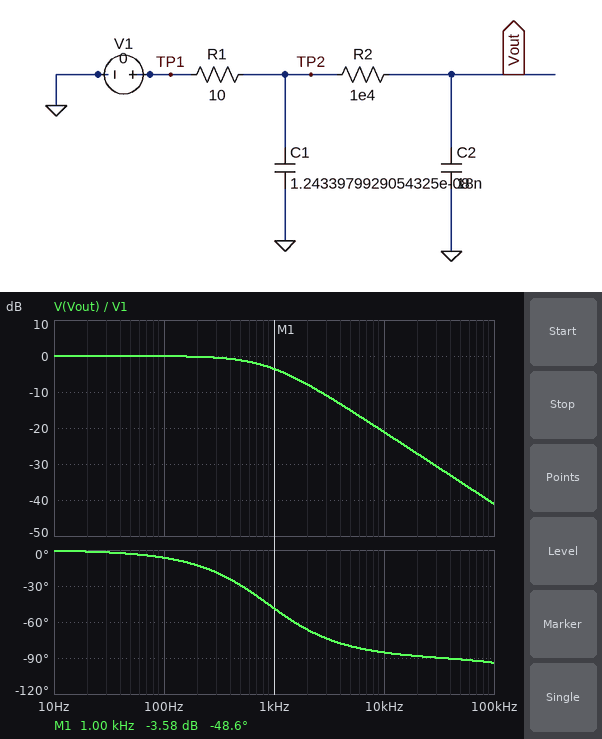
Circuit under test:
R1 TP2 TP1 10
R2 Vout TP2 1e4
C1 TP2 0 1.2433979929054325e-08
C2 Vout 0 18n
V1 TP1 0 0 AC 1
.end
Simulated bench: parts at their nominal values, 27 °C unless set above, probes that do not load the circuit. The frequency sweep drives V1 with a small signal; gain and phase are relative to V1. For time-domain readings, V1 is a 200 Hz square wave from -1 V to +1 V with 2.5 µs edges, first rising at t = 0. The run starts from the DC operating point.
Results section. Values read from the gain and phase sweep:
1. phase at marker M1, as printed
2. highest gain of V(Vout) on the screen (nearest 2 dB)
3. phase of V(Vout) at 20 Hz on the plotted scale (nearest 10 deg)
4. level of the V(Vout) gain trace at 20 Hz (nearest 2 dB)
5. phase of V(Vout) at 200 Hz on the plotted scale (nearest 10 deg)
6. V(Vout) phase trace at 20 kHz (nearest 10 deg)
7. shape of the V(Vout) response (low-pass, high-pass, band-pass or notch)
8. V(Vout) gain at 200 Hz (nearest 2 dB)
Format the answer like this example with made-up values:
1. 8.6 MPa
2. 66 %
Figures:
1. -48.6 deg
2. 0 dB
3. 0 deg
4. 0 dB
5. -10 deg
6. -90 deg
7. low-pass
8. 0 dB
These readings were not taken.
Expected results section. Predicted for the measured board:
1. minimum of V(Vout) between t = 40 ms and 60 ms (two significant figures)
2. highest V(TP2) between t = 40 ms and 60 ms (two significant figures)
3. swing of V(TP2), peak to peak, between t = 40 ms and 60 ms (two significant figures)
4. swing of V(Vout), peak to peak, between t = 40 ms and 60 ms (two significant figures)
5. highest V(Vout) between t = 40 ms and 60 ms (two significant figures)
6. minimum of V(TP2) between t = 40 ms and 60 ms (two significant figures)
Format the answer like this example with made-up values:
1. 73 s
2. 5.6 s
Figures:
1. -1.0 V
2. 1.0 V
3. 2.0 V
4. 2.0 V
5. 1.0 V
6. -1.0 V
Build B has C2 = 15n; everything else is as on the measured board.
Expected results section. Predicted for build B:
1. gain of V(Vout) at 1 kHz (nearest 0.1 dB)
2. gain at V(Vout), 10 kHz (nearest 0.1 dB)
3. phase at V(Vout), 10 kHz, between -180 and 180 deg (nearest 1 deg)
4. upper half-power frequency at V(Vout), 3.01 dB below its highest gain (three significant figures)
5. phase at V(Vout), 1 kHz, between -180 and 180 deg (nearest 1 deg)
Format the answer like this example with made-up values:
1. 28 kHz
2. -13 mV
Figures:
1. -2.8 dB
2. -19.5 dB
3. -84 deg
4. 1.06 kHz
5. -43 deg
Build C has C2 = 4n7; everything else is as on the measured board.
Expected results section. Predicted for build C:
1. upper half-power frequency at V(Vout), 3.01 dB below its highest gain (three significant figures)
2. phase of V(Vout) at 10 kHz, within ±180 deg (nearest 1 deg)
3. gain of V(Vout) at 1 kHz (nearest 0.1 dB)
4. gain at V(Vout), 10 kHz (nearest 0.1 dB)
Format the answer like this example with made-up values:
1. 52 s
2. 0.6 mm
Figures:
1. 3.38 kHz
2. -72 deg
3. -0.4 dB
4. -9.9 dB
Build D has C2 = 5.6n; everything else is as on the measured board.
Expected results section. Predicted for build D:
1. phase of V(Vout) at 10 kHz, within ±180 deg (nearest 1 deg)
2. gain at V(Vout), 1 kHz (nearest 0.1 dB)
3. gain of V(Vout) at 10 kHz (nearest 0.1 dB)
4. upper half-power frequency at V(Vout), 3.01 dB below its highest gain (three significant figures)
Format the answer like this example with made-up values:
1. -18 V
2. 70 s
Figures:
1. -75 deg
2. -0.5 dB
3. -11.3 dB
4. 2.84 kHz
